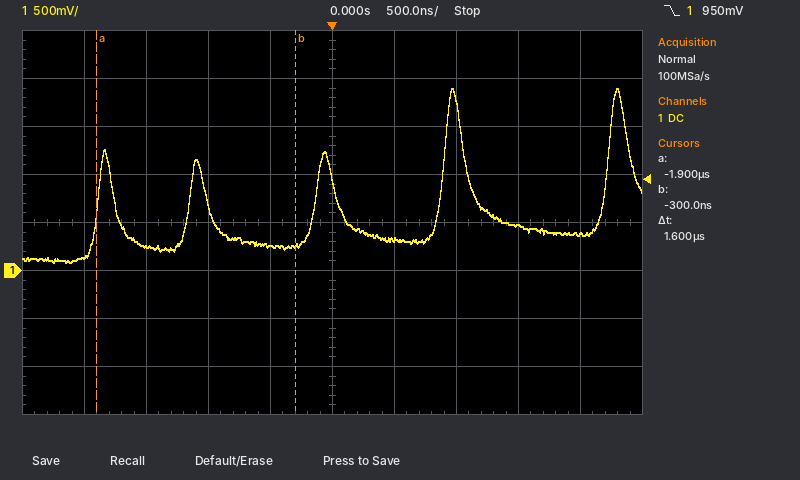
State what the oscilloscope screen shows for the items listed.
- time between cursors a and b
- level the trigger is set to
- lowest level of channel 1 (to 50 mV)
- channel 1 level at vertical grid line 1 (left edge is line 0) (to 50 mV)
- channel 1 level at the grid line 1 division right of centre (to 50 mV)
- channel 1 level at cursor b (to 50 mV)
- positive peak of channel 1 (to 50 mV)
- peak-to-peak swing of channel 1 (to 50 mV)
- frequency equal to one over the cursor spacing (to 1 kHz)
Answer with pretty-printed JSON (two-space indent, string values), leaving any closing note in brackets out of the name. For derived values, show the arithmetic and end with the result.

{
  "time between cursors a and b": "1.6 µs",
  "level the trigger is set to": "950 mV",
  "lowest level of channel 1": "100 mV",
  "channel 1 level at vertical grid line 1 (left edge is line 0)": "150 mV",
  "channel 1 level at the grid line 1 division right of centre": "300 mV",
  "channel 1 level at cursor b": "250 mV",
  "positive peak of channel 1": "1.90 V",
  "peak-to-peak swing of channel 1": "1.90 V − (100 mV) = 1.80 V",
  "frequency equal to one over the cursor spacing": "1 / 1.6 µs ≈ 625 kHz"
}
